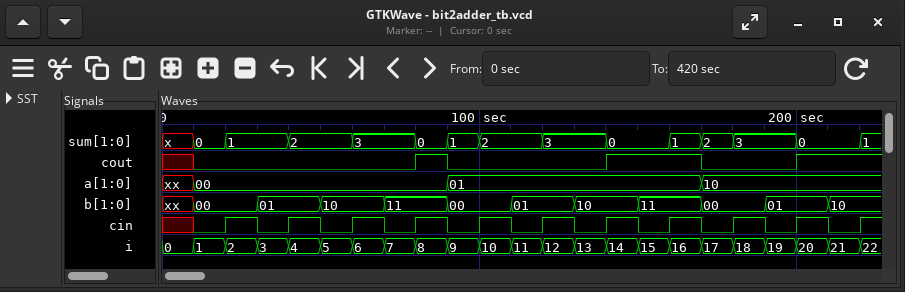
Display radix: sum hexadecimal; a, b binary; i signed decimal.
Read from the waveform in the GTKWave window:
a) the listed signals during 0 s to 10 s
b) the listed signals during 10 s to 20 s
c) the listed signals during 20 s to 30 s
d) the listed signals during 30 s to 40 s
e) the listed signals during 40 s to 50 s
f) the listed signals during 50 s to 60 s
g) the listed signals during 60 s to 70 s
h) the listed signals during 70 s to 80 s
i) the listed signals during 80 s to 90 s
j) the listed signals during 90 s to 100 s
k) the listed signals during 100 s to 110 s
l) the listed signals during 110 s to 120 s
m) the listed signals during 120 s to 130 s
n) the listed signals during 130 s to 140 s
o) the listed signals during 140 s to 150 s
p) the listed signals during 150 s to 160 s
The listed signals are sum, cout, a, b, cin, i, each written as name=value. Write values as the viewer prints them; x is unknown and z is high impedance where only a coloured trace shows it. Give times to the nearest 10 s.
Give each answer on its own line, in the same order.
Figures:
sum=x, cout=x, a=xx, b=xx, cin=x, i=0
sum=0, cout=0, a=00, b=00, cin=0, i=1
sum=1, cout=0, a=00, b=00, cin=1, i=2
sum=1, cout=0, a=00, b=01, cin=0, i=3
sum=2, cout=0, a=00, b=01, cin=1, i=4
sum=2, cout=0, a=00, b=10, cin=0, i=5
sum=3, cout=0, a=00, b=10, cin=1, i=6
sum=3, cout=0, a=00, b=11, cin=0, i=7
sum=0, cout=1, a=00, b=11, cin=1, i=8
sum=1, cout=0, a=01, b=00, cin=0, i=9
sum=2, cout=0, a=01, b=00, cin=1, i=10
sum=2, cout=0, a=01, b=01, cin=0, i=11
sum=3, cout=0, a=01, b=01, cin=1, i=12
sum=3, cout=0, a=01, b=10, cin=0, i=13
sum=0, cout=1, a=01, b=10, cin=1, i=14
sum=0, cout=1, a=01, b=11, cin=0, i=15
